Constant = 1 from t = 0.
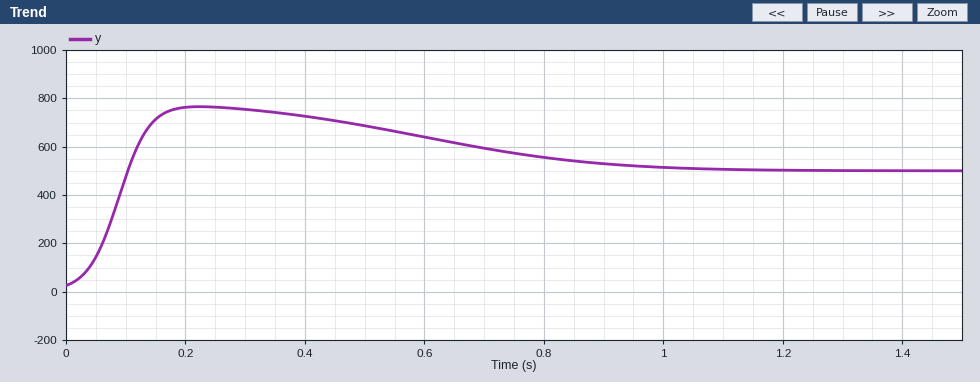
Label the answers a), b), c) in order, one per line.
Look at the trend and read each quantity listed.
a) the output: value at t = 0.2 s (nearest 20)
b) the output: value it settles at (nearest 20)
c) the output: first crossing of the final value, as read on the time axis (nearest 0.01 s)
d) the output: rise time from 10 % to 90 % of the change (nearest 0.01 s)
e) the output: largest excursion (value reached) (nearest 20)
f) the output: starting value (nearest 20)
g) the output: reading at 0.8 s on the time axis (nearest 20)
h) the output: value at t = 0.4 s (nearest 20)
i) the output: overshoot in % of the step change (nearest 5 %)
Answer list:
a) 760
b) 500
c) 0.10 s
d) 0.07 s
e) 760
f) 20
g) 560
h) 720
i) 55 %
